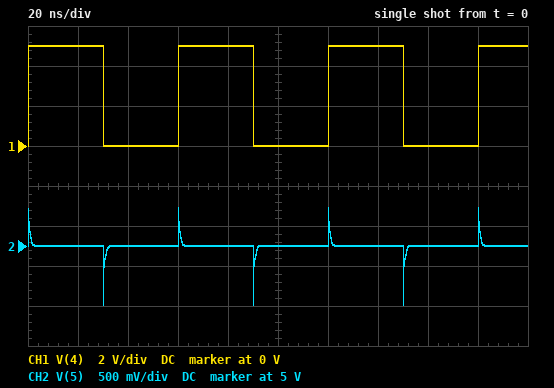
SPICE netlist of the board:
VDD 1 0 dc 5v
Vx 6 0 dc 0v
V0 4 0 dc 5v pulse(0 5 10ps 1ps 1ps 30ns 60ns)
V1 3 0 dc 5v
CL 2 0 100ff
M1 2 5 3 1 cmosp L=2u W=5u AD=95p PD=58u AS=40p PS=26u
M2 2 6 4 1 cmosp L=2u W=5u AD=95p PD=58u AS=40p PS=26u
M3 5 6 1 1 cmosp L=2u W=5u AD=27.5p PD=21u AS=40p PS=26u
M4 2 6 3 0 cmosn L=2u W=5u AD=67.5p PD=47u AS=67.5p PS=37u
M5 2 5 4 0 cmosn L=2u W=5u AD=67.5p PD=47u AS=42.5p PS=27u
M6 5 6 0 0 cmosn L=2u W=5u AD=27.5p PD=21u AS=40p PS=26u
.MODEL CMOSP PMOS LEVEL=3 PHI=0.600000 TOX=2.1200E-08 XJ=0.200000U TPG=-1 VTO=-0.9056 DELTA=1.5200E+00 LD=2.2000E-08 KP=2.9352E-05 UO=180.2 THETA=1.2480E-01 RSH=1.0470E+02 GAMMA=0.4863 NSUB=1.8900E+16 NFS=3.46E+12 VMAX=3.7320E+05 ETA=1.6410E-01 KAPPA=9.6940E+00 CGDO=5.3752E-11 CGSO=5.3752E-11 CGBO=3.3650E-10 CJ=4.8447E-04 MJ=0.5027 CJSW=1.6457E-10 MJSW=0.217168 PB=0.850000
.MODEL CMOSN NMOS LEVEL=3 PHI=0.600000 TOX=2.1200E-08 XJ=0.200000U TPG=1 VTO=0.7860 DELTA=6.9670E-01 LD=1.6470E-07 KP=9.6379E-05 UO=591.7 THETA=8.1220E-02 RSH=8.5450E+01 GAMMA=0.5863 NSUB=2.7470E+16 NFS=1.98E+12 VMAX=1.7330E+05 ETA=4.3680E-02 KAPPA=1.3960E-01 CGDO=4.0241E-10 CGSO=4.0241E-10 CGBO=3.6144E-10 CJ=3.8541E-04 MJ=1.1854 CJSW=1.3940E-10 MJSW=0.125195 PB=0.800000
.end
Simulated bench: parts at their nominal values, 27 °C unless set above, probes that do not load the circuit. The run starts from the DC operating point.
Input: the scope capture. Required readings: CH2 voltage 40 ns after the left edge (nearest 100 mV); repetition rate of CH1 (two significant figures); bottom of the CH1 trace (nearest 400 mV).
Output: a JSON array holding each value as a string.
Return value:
["5.0 V", "17 MHz", "0 V"]
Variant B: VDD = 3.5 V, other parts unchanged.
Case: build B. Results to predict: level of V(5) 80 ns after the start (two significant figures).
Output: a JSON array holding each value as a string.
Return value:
["3.5 V"]
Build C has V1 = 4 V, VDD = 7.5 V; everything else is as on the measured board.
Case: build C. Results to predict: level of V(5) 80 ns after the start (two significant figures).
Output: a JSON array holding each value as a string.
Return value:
["7.5 V"]
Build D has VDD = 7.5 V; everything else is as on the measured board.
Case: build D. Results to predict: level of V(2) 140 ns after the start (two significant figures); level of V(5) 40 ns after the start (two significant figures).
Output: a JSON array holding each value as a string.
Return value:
["5.0 V", "7.5 V"]
